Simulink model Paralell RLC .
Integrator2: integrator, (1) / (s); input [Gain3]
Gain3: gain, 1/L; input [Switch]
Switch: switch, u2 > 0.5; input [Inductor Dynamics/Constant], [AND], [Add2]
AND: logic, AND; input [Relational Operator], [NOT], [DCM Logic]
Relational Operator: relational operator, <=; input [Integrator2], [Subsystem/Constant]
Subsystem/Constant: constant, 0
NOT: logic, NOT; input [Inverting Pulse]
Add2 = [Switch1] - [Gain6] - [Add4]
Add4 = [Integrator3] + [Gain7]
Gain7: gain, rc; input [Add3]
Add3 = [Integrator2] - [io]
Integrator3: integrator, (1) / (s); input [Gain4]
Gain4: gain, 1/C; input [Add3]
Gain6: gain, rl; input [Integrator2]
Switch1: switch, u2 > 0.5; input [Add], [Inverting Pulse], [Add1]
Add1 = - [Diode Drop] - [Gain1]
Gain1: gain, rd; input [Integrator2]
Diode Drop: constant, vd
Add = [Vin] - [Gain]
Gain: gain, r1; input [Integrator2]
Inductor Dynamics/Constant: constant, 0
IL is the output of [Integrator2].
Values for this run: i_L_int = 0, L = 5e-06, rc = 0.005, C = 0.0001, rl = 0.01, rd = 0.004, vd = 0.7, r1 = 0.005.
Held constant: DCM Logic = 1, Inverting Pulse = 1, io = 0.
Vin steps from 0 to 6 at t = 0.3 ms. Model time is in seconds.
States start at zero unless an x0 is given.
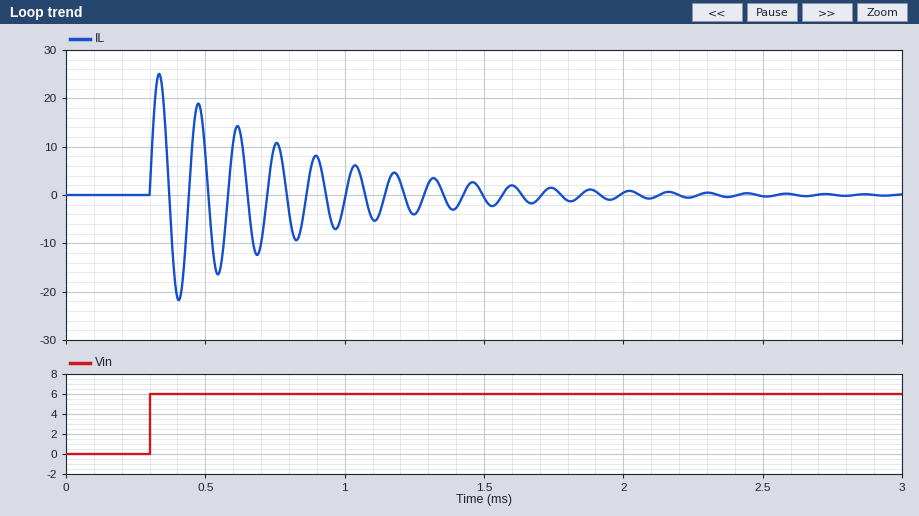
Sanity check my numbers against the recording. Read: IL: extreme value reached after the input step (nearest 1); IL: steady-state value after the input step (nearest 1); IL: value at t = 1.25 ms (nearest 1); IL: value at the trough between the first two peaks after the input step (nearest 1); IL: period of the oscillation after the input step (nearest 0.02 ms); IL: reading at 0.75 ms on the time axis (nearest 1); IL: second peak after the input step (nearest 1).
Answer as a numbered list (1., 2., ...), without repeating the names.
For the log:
1. 25
2. 0
3. -4
4. -22
5. 0.14 ms
6. 10
7. 19
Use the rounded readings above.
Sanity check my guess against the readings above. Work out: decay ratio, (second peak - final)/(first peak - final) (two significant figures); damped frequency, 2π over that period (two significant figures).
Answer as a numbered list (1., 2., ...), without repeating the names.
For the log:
1. 0.76
2. 45 rad/ms
